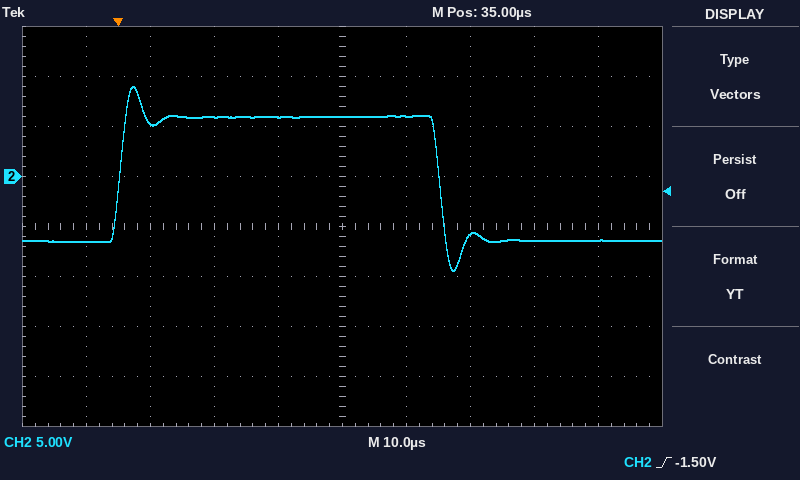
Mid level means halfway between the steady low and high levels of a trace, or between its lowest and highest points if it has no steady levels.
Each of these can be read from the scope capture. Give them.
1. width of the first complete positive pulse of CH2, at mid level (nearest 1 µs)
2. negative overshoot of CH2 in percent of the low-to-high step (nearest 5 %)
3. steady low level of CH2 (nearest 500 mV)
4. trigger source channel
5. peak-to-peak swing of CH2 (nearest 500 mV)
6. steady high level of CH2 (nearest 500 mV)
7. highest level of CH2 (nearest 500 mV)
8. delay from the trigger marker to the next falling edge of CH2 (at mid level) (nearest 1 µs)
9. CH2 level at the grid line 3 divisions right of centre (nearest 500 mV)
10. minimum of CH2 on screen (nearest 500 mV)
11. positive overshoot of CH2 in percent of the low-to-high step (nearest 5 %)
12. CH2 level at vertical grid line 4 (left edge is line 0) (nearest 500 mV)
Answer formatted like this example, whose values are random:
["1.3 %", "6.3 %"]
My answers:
["50 µs", "25 %", "-6.5 V", "CH2", "18.5 V", "6.0 V", "9.0 V", "50 µs", "-6.5 V", "-9.5 V", "25 %", "6.0 V"]
